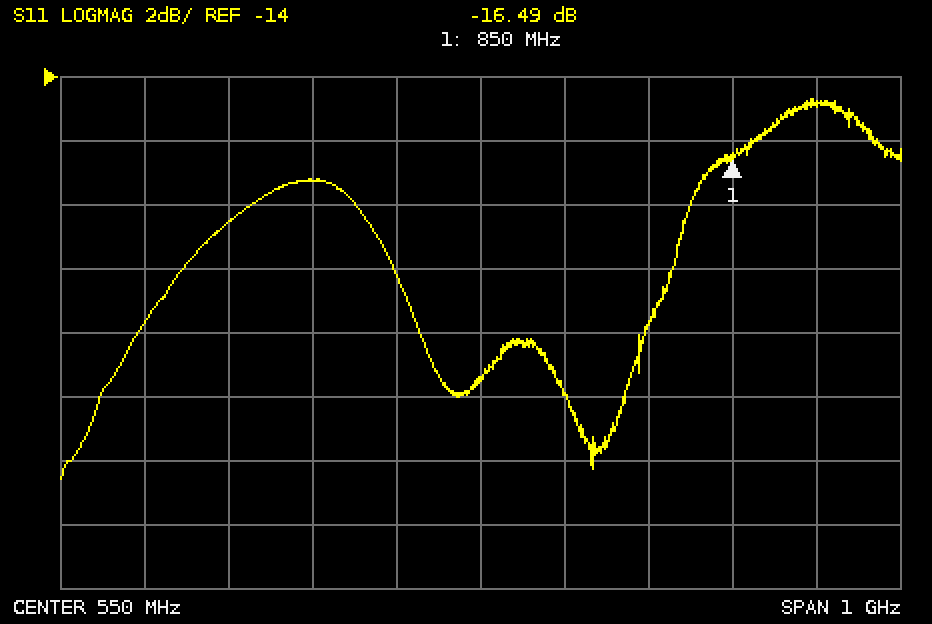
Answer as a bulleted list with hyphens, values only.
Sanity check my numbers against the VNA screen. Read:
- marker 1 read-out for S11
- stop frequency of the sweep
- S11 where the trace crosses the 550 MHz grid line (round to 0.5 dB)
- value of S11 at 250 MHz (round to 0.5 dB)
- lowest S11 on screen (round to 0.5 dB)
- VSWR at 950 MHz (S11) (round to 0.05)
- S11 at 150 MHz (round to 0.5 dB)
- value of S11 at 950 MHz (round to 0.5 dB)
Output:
- -16.49 dB
- 1.05 GHz
- -23.5 dB
- -18.5 dB
- -26.5 dB
- 1.45
- -21.5 dB
- -15.0 dB
